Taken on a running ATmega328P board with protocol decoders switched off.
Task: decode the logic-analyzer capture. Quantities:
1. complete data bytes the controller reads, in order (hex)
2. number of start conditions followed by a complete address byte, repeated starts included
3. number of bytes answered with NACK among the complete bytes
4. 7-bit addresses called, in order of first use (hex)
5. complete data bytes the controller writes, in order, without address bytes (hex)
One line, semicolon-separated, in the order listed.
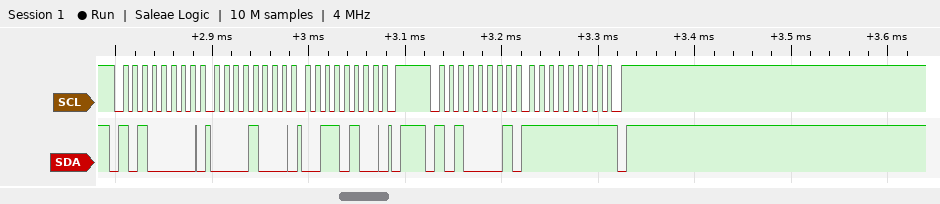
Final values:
FF; 2; 1; 0x50; 08 34
